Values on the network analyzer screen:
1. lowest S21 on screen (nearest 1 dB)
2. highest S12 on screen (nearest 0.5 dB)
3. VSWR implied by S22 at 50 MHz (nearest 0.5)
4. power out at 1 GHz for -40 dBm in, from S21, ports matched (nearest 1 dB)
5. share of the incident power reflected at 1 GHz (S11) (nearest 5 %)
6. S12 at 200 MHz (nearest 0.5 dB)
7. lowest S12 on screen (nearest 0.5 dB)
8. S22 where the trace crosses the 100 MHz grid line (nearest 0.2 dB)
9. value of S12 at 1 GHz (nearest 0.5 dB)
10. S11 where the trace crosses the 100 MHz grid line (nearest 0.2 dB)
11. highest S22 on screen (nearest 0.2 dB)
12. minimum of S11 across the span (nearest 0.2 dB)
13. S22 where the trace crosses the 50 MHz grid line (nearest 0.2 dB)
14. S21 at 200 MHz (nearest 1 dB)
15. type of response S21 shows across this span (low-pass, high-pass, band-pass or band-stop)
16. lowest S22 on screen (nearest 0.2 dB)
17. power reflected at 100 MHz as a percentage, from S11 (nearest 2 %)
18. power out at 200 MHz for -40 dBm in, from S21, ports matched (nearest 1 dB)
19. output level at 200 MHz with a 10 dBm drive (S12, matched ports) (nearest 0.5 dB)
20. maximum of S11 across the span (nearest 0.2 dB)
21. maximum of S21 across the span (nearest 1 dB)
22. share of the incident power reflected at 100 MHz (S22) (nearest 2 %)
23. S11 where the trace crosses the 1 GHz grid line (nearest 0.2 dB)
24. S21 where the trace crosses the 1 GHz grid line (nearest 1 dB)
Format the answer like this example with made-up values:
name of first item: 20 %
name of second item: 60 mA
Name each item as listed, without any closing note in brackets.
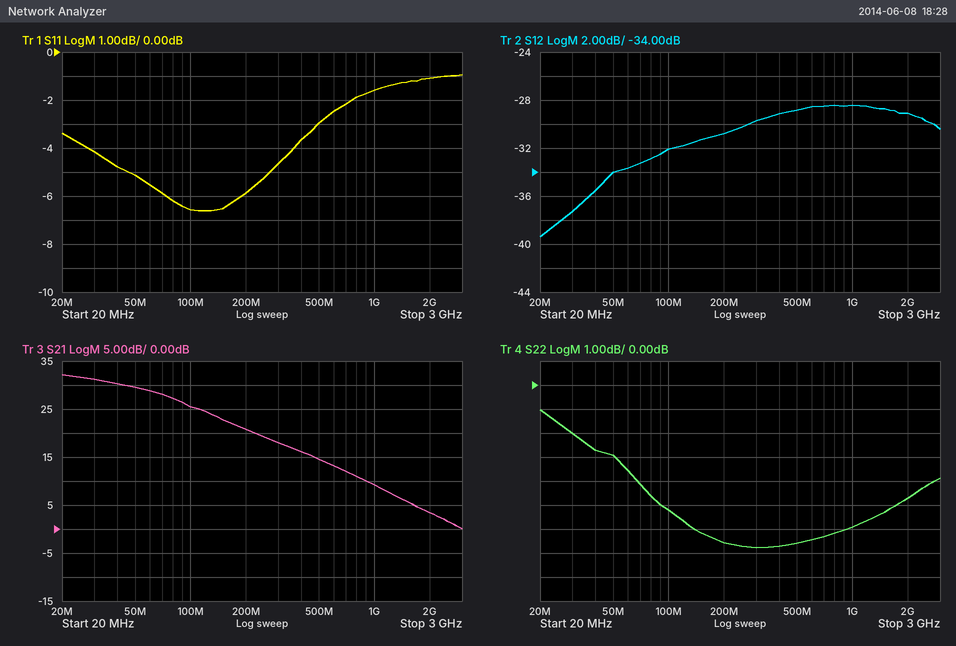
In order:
lowest S21 on screen: 0 dB
highest S12 on screen: -28.5 dB
VSWR implied by S22 at 50 MHz: 6.0
power out at 1 GHz for -40 dBm in, from S21, ports matched: -31 dBm
share of the incident power reflected at 1 GHz (S11): 70 %
S12 at 200 MHz: -31.0 dB
lowest S12 on screen: -39.5 dB
S22 where the trace crosses the 100 MHz grid line: -5.2 dB
value of S12 at 1 GHz: -28.5 dB
S11 where the trace crosses the 100 MHz grid line: -6.6 dB
highest S22 on screen: -1.0 dB
minimum of S11 across the span: -6.6 dB
S22 where the trace crosses the 50 MHz grid line: -3.0 dB
S21 at 200 MHz: 21 dB
type of response S21 shows across this span: low-pass
lowest S22 on screen: -6.8 dB
power reflected at 100 MHz as a percentage, from S11: 22 %
power out at 200 MHz for -40 dBm in, from S21, ports matched: -19 dBm
output level at 200 MHz with a 10 dBm drive (S12, matched ports): -21.0 dBm
maximum of S11 across the span: -1.0 dB
maximum of S21 across the span: 32 dB
share of the incident power reflected at 100 MHz (S22): 30 %
S11 where the trace crosses the 1 GHz grid line: -1.6 dB
S21 where the trace crosses the 1 GHz grid line: 9 dB
